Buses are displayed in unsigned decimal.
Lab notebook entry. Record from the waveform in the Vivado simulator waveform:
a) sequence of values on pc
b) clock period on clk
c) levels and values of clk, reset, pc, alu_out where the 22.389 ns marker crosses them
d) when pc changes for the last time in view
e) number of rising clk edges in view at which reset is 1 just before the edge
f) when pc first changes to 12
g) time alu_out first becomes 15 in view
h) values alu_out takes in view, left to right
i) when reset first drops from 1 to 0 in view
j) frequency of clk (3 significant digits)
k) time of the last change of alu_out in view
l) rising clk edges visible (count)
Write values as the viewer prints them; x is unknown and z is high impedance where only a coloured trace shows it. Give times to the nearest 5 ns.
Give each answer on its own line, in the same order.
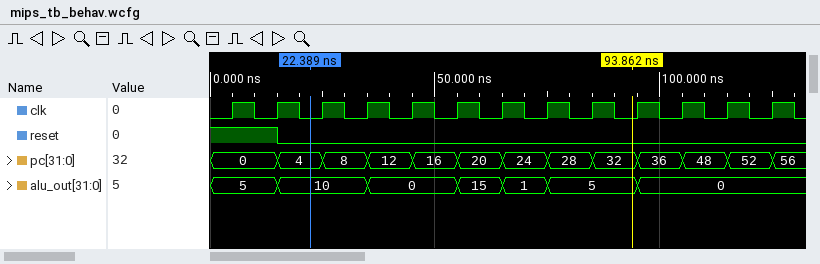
0, 4, 8, 12, 16, 20, 24, 28, 32, 36, 48, 52, 56
10 ns
clk=0, reset=0, pc=4, alu_out=10
125 ns
2
35 ns
55 ns
5, 10, 0, 15, 1, 5, 0
15 ns
100 MHz
95 ns
13
